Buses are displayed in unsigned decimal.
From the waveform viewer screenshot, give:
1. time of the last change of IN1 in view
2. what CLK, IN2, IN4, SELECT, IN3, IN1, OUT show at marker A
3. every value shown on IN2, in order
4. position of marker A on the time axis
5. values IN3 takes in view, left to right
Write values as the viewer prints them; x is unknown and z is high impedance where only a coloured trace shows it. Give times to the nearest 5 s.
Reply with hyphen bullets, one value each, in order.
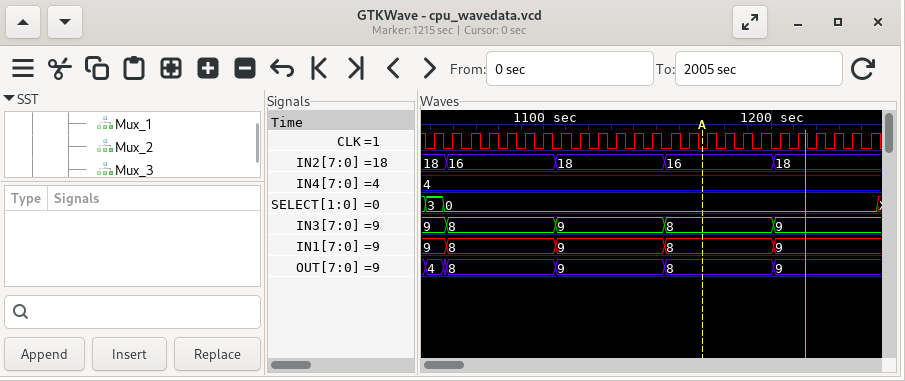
- 1200 s
- CLK=0, IN2=16, IN4=4, SELECT=0, IN3=8, IN1=8, OUT=8
- 18, 16, 18, 16, 18
- 1170 s
- 9, 8, 9, 8, 9
